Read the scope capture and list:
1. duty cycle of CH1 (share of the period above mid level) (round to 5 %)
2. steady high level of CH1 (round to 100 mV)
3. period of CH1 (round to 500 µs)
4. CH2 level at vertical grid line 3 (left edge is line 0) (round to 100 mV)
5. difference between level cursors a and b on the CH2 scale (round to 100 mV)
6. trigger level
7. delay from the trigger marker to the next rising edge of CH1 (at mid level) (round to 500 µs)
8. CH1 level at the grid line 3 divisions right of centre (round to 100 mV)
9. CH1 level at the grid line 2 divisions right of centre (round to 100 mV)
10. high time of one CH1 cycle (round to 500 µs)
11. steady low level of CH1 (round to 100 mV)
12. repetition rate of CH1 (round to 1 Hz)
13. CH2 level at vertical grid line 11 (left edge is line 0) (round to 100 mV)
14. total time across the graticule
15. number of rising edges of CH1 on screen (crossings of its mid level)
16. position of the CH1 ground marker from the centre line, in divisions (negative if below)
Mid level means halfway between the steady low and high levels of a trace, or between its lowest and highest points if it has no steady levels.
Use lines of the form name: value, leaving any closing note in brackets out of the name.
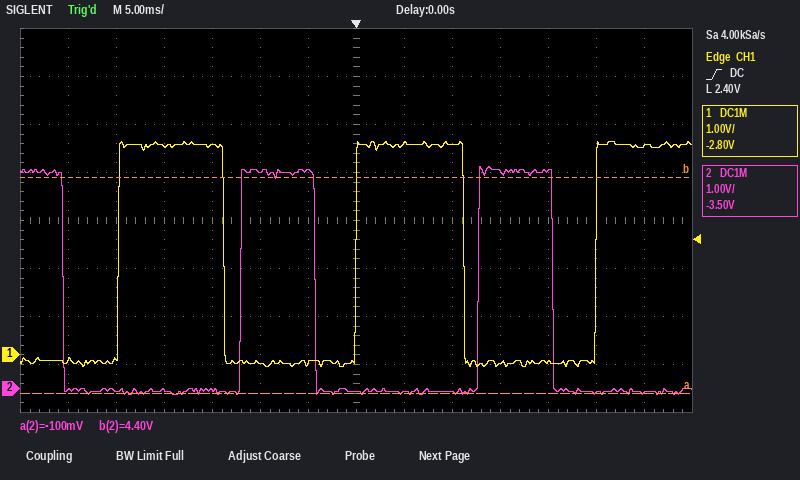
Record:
duty cycle of CH1 (share of the period above mid level): 45 %
steady high level of CH1: 4.4 V
period of CH1: 25.0 ms
CH2 level at vertical grid line 3 (left edge is line 0): 0.0 V
difference between level cursors a and b on the CH2 scale: 4.5 V
trigger level: 2.40 V
delay from the trigger marker to the next rising edge of CH1 (at mid level): 25.0 ms
CH1 level at the grid line 3 divisions right of centre: -200 mV
CH1 level at the grid line 2 divisions right of centre: 4.4 V
high time of one CH1 cycle: 11.0 ms
steady low level of CH1: -200 mV
repetition rate of CH1: 40 Hz
CH2 level at vertical grid line 11 (left edge is line 0): 4.5 V
total time across the graticule: 70 ms
number of rising edges of CH1 on screen: 3
position of the CH1 ground marker from the centre line, in divisions: -2.8 div
